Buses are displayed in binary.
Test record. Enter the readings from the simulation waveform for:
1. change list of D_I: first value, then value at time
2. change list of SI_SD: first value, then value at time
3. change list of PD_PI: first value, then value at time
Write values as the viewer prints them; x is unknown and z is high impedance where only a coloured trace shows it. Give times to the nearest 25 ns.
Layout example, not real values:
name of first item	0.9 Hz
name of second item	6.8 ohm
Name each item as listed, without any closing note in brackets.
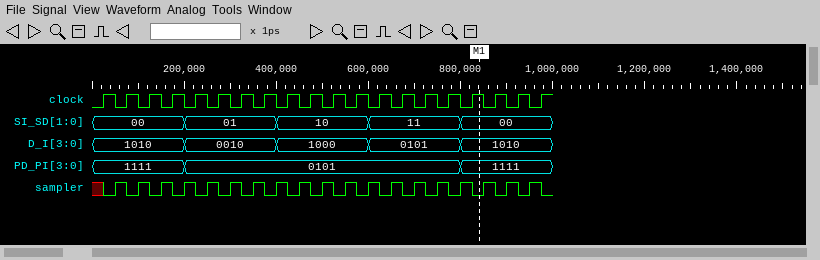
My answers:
change list of D_I: first value, then value at time	1010, 0010 at 200 ns, 1000 at 400 ns, 0101 at 600 ns, 1010 at 800 ns
change list of SI_SD: first value, then value at time	00, 01 at 200 ns, 10 at 400 ns, 11 at 600 ns, 00 at 800 ns
change list of PD_PI: first value, then value at time	1111, 0101 at 200 ns, 1111 at 800 ns
